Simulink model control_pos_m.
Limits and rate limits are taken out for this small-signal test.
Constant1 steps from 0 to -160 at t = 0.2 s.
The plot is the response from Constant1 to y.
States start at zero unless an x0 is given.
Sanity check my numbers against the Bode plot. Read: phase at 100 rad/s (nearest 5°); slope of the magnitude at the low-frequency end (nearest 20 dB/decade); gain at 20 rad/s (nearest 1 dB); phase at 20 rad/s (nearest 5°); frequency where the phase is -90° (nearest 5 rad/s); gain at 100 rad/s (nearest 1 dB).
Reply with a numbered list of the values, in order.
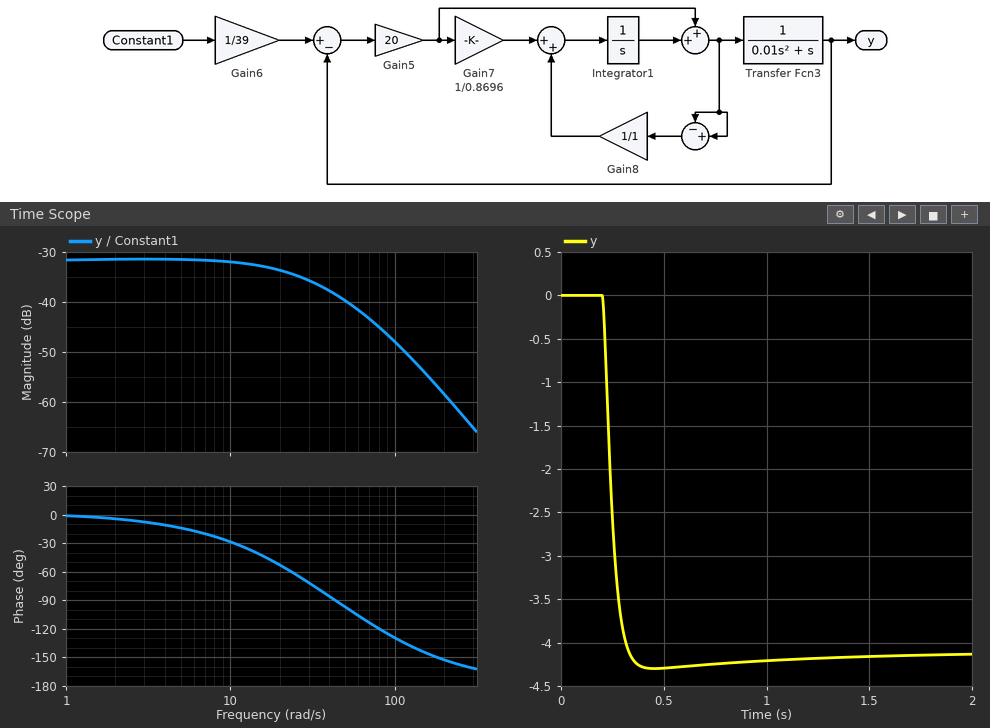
1. -130°
2. 0 dB/decade
3. -34 dB
4. -55°
5. 45 rad/s
6. -48 dB
